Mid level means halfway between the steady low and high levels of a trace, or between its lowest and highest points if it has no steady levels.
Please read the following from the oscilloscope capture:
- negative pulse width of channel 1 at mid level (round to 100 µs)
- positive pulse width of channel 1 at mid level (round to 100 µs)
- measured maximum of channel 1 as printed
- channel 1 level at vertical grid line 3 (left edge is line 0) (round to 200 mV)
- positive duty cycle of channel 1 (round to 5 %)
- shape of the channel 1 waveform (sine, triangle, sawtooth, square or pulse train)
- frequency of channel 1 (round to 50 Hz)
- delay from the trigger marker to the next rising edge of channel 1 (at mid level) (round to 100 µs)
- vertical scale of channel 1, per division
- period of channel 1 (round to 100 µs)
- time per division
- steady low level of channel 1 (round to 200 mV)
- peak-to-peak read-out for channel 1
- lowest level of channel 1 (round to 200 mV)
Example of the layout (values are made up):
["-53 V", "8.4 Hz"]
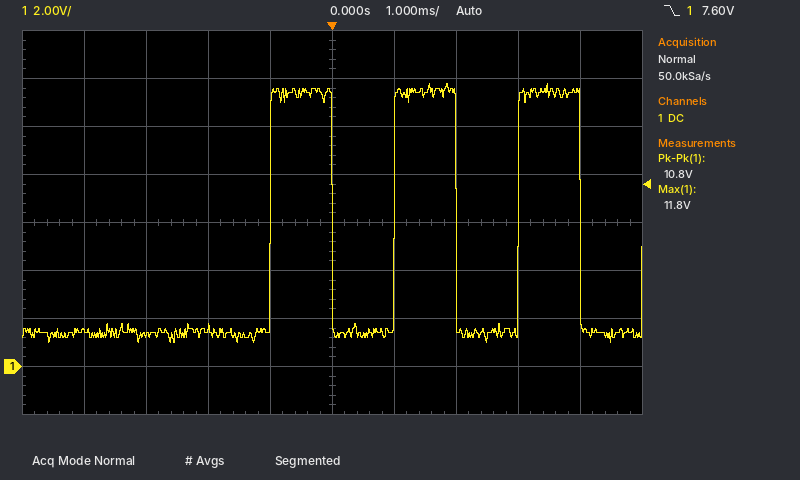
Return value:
["1.0 ms", "1.0 ms", "11.8 V", "1.6 V", "50 %", "square", "500 Hz", "1.0 ms", "2 V", "2.0 ms", "1 ms", "1.4 V", "10.8 V", "1.0 V"]
